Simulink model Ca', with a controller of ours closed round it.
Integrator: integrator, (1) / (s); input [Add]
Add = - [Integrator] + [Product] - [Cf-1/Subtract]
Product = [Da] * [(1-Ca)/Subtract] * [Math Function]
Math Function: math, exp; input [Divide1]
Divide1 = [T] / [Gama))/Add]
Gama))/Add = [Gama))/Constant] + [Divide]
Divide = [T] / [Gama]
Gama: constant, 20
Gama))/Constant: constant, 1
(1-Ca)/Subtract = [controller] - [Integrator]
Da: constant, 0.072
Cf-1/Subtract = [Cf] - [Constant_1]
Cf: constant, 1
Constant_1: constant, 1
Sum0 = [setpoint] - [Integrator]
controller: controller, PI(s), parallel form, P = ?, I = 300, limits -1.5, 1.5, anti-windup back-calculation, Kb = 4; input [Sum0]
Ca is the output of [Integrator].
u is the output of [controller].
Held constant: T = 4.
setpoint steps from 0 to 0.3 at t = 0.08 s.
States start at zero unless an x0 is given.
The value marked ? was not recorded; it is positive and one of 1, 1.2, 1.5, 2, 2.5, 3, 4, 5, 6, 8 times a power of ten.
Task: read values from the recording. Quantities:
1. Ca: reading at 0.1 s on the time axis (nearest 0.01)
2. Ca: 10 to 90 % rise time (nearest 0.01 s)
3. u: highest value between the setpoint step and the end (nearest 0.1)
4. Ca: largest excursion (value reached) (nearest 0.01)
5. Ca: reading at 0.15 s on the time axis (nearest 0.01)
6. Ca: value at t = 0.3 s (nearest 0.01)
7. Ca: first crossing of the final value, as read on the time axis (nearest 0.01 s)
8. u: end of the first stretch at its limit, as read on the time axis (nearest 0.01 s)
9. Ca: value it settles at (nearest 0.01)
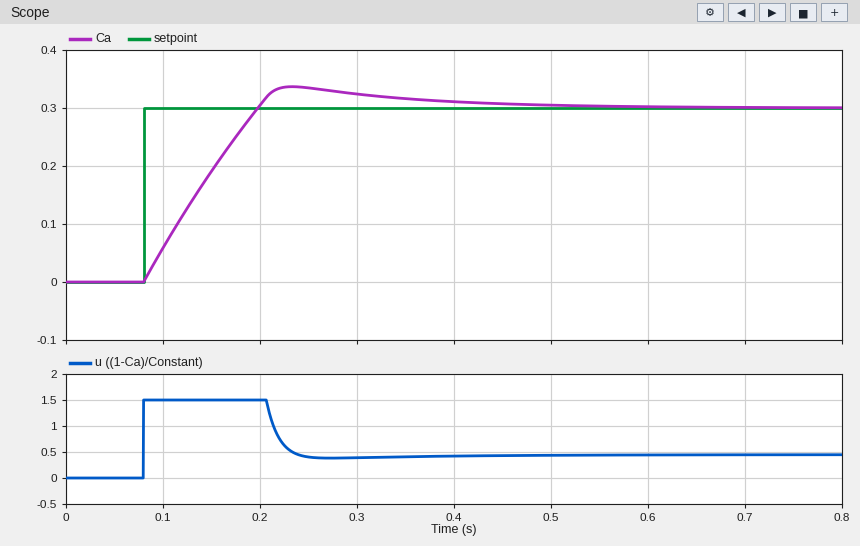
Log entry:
0.06
0.09 s
1.5
0.34
0.19
0.32
0.20 s
0.21 s
0.30
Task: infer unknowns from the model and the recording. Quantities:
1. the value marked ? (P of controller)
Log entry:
40
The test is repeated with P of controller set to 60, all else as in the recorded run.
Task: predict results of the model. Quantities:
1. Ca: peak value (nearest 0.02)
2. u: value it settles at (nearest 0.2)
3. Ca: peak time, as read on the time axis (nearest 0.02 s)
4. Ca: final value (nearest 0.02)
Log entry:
0.32
0.4
0.22 s
0.30
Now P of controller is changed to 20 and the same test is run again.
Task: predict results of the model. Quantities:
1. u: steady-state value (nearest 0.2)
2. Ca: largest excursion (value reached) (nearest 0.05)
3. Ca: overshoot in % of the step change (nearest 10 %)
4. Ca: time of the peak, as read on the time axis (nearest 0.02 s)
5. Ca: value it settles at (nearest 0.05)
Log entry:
0.4
0.40
30 %
0.26 s
0.30
